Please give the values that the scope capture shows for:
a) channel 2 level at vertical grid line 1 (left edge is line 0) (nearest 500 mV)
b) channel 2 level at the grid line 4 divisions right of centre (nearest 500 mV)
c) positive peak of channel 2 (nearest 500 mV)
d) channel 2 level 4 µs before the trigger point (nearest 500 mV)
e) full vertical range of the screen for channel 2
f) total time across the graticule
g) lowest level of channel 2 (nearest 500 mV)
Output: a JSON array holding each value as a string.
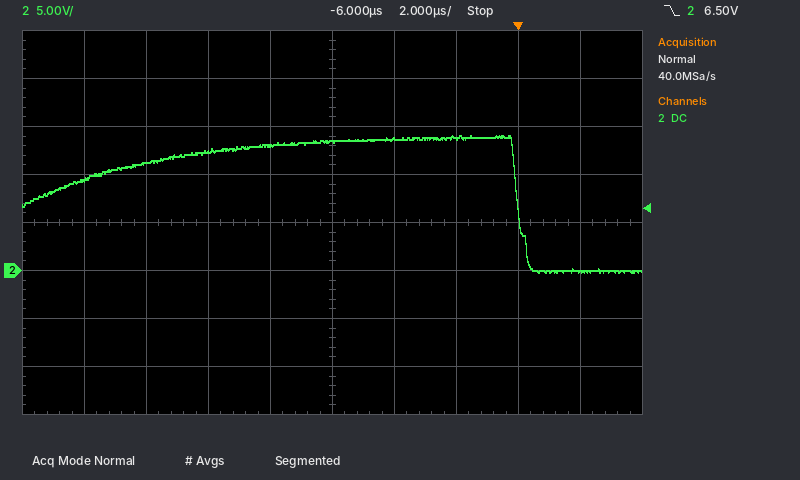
["9.5 V", "0.0 V", "14.0 V", "13.5 V", "40 V", "20 µs", "0.0 V"]
